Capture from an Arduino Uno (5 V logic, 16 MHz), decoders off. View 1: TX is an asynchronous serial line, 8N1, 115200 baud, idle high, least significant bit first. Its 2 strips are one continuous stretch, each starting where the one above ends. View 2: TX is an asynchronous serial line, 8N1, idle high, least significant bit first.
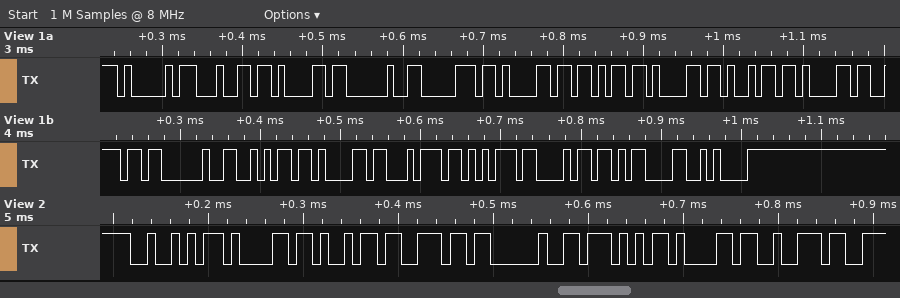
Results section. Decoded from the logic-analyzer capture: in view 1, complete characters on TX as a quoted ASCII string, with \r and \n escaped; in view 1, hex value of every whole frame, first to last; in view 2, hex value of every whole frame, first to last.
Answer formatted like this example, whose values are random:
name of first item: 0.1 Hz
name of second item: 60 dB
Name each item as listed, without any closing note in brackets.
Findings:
in view 1, complete characters on TX as a quoted ASCII string, with \r and \n escaped: "Ada pakaian jatuh\r\n"
in view 1, hex value of every whole frame, first to last: 0x41 0x64 0x61 0x20 0x70 0x61 0x6B 0x61 0x69 0x61 0x6E 0x20 0x6A 0x61 0x74 0x75 0x68 0x0D 0x0A
in view 2, hex value of every whole frame, first to last: 0x52 0x61 0x69 0x6E 0x20 0x57 0x61 0x72
